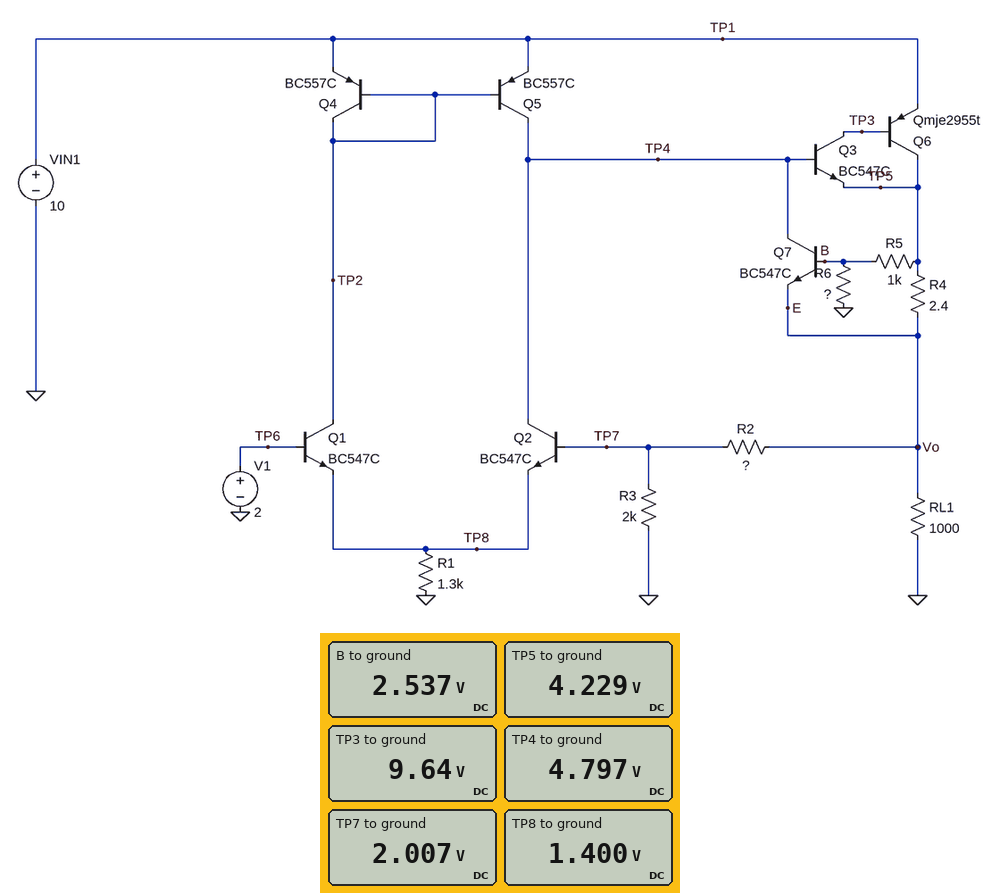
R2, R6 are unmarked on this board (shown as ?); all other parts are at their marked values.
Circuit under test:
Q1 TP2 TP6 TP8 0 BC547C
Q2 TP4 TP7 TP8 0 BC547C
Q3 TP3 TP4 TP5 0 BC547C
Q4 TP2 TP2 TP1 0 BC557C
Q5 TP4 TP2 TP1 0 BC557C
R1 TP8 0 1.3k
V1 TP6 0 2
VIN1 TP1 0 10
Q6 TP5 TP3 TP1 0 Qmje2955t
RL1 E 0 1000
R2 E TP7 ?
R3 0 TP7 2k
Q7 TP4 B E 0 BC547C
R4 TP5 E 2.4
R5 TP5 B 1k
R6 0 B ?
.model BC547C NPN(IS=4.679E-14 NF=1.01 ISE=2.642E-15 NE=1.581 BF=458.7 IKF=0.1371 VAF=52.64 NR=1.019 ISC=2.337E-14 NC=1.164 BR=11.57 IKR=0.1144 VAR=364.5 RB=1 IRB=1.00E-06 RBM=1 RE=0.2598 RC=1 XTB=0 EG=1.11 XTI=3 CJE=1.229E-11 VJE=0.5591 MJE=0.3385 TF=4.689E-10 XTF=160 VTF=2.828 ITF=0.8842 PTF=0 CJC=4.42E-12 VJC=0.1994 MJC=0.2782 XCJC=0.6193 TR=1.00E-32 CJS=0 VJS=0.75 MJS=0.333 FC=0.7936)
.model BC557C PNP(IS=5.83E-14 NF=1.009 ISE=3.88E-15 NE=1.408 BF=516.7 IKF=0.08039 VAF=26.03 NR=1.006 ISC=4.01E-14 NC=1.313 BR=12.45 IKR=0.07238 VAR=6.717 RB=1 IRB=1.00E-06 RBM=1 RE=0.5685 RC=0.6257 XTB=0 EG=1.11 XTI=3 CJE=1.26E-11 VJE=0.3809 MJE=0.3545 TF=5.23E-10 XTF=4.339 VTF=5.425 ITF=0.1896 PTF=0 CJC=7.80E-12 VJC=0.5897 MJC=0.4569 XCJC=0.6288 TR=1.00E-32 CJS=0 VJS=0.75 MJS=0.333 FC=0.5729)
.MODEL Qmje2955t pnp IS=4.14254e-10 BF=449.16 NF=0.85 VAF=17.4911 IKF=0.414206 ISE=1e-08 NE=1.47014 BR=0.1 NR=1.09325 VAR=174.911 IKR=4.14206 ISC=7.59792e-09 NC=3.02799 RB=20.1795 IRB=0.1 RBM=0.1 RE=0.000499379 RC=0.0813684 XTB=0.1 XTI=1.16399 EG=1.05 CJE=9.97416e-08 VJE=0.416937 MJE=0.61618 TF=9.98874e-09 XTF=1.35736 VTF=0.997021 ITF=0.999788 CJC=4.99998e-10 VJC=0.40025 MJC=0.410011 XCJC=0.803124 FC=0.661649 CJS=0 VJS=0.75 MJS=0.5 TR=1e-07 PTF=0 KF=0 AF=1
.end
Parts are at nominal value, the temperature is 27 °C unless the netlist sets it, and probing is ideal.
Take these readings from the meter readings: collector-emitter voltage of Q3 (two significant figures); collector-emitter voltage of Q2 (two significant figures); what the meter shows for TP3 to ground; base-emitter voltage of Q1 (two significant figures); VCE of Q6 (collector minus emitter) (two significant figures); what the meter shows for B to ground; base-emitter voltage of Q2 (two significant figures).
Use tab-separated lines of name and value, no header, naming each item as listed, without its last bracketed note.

collector-emitter voltage of Q3	5.4 V
collector-emitter voltage of Q2	3.4 V
what the meter shows for TP3 to ground	9.64 V
base-emitter voltage of Q1	600 mV
VCE of Q6 (collector minus emitter)	-5.8 V
what the meter shows for B to ground	2.537 V
base-emitter voltage of Q2	610 mV
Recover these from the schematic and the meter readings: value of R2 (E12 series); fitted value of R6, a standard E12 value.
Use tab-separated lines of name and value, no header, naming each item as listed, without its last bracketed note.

value of R2	2.2 kΩ
fitted value of R6, a standard E12 value	1.5 kΩ
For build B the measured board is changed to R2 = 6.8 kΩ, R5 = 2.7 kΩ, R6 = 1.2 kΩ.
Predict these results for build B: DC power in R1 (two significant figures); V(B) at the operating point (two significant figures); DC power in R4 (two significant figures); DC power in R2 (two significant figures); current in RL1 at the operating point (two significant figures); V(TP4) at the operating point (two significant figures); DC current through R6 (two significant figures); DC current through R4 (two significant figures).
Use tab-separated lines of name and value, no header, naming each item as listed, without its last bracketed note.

DC power in R1	1.5 mW
V(B) at the operating point	2.7 V
DC power in R4	230 µW
DC power in R2	6.8 mW
current in RL1 at the operating point	8.8 mA
V(TP4) at the operating point	9.4 V
DC current through R6	2.3 mA
DC current through R4	9.8 mA
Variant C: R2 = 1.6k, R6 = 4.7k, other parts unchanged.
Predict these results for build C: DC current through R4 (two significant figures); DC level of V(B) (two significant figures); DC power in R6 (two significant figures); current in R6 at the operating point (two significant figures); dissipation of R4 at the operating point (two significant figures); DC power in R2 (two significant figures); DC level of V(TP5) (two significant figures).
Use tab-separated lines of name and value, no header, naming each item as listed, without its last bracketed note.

DC current through R4	4.6 mA
DC level of V(B)	3.0 V
DC power in R6	1.9 mW
current in R6 at the operating point	640 µA
dissipation of R4 at the operating point	51 µW
DC power in R2	1.6 mW
DC level of V(TP5)	3.6 V
